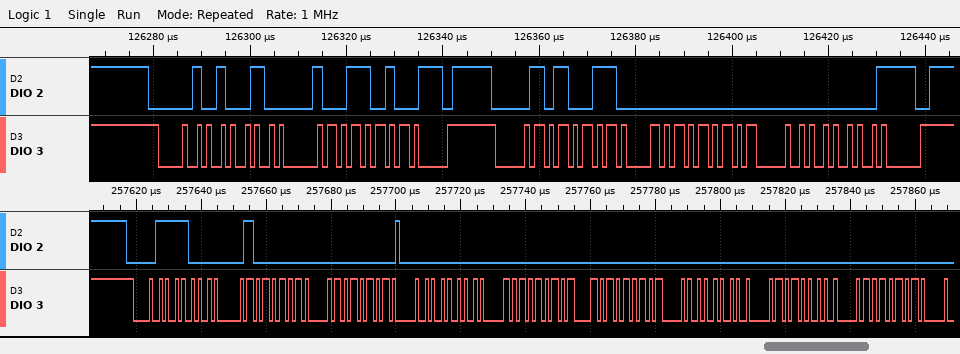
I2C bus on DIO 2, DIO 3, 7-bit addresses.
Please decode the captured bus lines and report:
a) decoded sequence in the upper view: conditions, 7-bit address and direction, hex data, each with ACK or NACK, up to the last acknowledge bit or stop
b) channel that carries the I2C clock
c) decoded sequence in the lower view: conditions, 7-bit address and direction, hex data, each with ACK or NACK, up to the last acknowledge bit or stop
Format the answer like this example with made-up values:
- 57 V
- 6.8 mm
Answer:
- start, address 29 write ACK, 9A ACK, stop, start, address 29 read ACK, 00 ACK, 00 NACK, stop
- DIO 3
- start, address 3C write ACK, 40 ACK, 00 ACK, 00 ACK, 00 ACK, 00 ACK, 00 ACK, 00 ACK, 00 ACK
